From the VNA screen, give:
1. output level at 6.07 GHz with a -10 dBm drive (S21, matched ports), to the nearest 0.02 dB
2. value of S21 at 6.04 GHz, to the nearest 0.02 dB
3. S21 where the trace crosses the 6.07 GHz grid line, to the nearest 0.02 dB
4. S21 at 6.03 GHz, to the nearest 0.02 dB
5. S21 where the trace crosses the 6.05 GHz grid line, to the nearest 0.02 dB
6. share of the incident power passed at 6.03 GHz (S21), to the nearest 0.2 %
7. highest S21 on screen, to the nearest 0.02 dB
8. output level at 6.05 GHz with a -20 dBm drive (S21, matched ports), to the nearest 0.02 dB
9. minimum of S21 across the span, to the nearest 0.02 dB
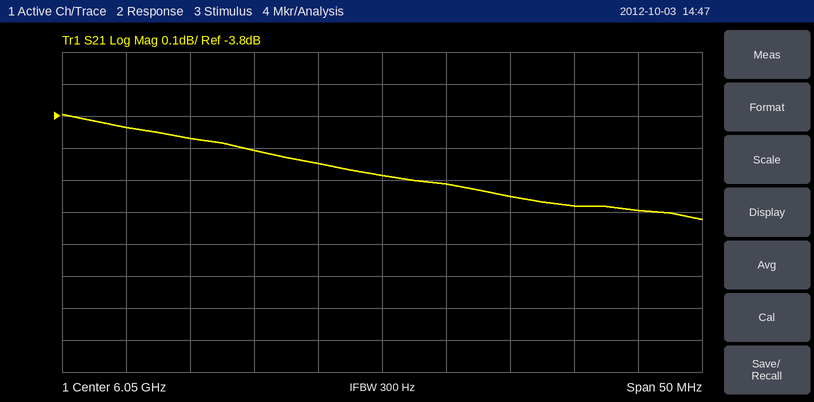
-14.10 dBm
-3.90 dB
-4.10 dB
-3.84 dB
-3.98 dB
41.4 %
-3.80 dB
-23.98 dBm
-4.12 dB
